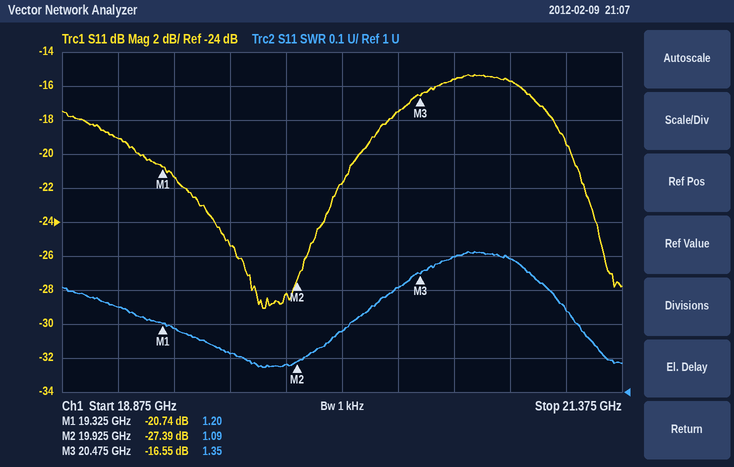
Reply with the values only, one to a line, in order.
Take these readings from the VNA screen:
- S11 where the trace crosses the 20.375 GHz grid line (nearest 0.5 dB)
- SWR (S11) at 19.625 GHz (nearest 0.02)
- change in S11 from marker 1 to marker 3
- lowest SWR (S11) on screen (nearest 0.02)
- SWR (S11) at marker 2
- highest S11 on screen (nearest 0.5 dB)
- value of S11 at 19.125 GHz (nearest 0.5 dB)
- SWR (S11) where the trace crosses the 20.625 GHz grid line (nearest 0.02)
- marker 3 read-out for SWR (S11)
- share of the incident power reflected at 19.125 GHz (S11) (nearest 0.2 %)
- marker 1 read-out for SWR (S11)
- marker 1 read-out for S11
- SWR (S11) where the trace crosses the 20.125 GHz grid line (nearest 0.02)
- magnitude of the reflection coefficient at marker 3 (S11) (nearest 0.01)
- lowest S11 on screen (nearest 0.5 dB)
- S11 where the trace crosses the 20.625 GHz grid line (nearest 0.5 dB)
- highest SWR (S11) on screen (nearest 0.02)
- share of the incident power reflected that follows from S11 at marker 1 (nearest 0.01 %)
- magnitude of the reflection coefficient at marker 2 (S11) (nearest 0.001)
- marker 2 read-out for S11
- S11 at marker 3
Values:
-17.5 dB
1.12
4.19 dB
1.08
1.09
-15.5 dB
-19.0 dB
1.40
1.35
1.2 %
1.20
-20.74 dB
1.18
0.15
-29.0 dB
-15.5 dB
1.42
0.84 %
0.043
-27.39 dB
-16.55 dB
